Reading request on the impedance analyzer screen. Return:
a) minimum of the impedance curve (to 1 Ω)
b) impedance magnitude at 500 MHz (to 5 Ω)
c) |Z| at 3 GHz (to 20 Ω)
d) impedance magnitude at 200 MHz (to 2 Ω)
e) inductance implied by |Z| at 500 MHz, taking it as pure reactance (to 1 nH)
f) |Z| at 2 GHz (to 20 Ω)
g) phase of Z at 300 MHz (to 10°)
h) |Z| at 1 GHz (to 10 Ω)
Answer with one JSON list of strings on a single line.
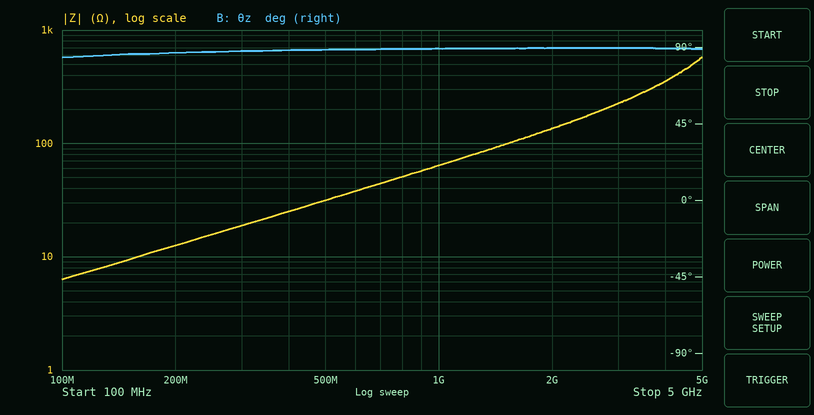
["6 Ω", "30 Ω", "220 Ω", "12 Ω", "10 nH", "140 Ω", "90°", "60 Ω"]
